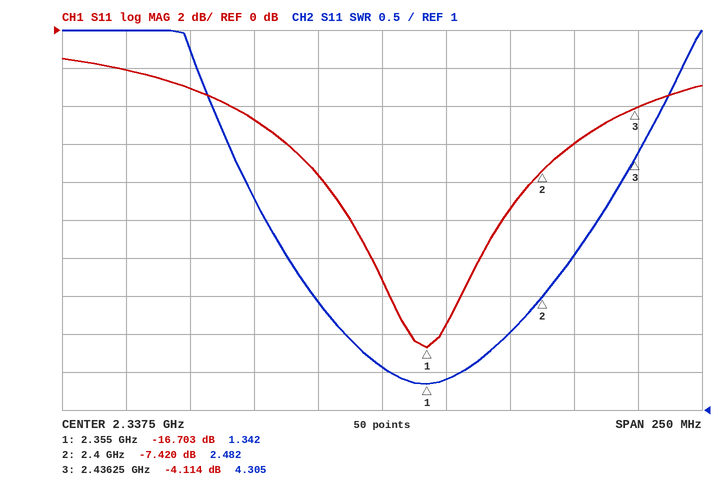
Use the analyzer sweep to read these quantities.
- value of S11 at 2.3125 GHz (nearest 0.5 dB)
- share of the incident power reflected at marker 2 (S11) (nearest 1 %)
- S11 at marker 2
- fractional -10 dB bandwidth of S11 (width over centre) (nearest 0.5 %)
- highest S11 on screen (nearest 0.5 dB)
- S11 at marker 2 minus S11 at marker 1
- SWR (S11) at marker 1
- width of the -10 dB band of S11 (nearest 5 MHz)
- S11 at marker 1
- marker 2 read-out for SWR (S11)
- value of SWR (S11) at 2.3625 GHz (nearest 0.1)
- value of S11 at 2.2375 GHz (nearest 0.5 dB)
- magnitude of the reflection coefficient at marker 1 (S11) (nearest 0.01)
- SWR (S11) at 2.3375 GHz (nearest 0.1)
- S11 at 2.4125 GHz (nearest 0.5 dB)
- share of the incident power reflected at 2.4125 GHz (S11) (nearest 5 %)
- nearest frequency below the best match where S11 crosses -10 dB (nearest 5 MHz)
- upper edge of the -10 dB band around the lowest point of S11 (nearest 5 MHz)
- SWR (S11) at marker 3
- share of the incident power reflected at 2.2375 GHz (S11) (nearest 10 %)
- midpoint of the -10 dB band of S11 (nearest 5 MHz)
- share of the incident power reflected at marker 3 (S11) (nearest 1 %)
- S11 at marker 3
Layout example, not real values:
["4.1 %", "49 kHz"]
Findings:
["-7.5 dB", "18 %", "-7.420 dB", "2.5 %", "-1.5 dB", "9.283 dB", "1.342", "60 MHz", "-16.703 dB", "2.482", "1.4", "-2.0 dB", "0.15", "1.6", "-6.0 dB", "25 %", "2.325 GHz", "2.385 GHz", "4.305", "60 %", "2.355 GHz", "39 %", "-4.114 dB"]
